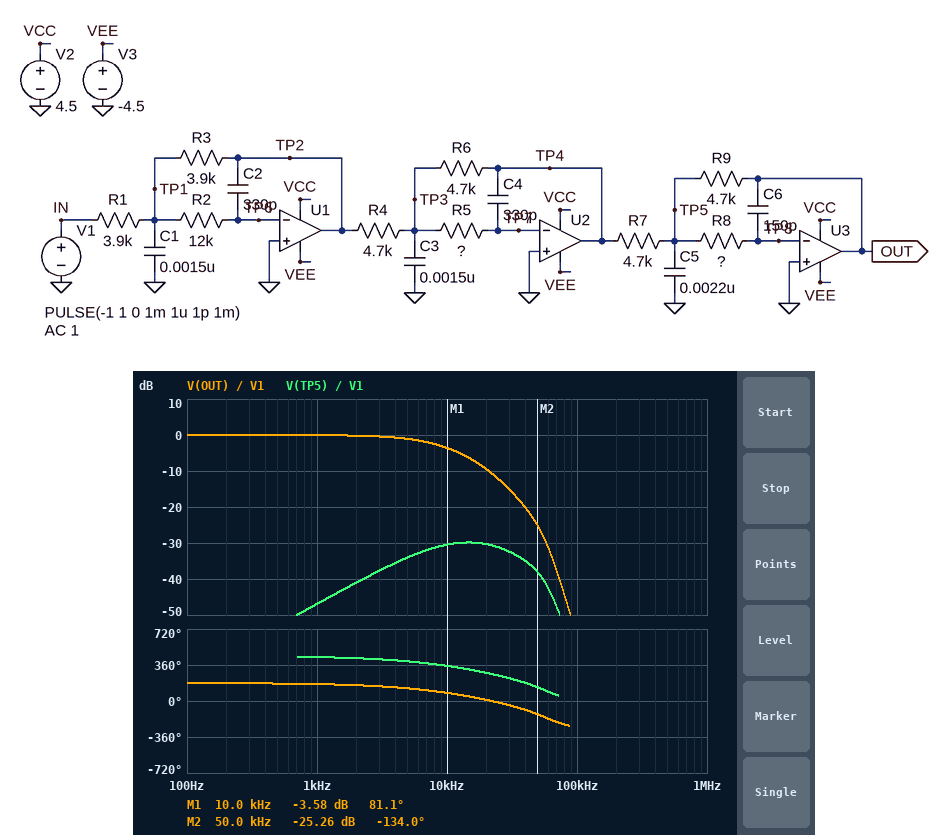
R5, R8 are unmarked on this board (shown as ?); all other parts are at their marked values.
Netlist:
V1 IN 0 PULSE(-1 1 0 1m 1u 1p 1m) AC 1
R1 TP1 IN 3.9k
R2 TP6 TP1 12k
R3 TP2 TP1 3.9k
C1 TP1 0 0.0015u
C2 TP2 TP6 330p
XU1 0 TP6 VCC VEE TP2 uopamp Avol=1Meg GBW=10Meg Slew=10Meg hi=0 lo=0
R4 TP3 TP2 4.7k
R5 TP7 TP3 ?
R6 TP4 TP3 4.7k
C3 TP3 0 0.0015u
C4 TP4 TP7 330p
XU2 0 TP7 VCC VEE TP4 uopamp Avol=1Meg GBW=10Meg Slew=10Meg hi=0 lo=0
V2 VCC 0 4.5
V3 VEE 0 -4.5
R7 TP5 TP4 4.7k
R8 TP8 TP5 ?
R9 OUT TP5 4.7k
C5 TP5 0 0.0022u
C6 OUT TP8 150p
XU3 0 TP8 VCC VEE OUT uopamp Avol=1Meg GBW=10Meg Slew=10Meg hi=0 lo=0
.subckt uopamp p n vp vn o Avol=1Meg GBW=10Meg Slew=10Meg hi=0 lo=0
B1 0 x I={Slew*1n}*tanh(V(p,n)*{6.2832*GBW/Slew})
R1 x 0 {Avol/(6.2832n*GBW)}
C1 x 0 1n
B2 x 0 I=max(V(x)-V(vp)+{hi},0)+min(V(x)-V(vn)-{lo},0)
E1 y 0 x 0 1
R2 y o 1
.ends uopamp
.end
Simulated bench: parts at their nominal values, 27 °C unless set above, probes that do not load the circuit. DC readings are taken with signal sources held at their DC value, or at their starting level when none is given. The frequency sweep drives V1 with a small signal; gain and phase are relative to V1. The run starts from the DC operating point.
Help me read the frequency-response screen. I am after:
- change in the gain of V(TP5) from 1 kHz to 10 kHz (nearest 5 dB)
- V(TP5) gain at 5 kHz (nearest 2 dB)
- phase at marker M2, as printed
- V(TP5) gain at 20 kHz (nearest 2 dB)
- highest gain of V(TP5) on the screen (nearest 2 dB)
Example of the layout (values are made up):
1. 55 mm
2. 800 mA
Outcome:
1. 15 dB
2. -34 dB
3. -134.0 deg
4. -30 dB
5. -30 dB
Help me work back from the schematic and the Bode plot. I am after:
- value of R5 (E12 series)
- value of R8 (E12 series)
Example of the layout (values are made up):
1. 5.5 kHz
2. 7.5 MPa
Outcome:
1. 27 kΩ
2. 4.7 kΩ
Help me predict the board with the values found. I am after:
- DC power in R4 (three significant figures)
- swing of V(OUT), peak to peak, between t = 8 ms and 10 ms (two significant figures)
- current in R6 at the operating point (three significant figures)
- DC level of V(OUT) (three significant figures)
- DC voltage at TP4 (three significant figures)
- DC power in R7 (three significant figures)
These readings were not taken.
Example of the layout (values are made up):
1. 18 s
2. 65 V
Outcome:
1. 213 µW
2. 1.8 V
3. 213 µA
4. 1.00 V
5. -1.00 V
6. 213 µW
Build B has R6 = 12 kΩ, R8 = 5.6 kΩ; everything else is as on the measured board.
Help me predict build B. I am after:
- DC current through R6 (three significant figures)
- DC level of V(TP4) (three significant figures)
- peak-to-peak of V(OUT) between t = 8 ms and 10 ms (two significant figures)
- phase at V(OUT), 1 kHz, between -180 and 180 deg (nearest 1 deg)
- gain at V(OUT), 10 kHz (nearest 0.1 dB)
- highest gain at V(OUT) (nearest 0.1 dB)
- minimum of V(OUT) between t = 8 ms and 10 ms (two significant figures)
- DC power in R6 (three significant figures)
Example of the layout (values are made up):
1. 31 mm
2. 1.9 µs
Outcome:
1. 213 µA
2. -2.55 V
3. 4.3 V
4. 163 deg
5. 0.6 dB
6. 8.1 dB
7. -2.3 V
8. 543 µW
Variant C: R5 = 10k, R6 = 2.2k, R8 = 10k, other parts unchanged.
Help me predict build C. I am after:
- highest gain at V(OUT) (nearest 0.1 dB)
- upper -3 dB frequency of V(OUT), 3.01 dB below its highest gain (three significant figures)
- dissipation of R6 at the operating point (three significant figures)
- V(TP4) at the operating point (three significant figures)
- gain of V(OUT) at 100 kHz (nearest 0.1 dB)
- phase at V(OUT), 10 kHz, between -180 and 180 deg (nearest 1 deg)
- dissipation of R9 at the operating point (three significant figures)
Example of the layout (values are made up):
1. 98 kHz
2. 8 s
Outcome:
1. -6.6 dB
2. 24.0 kHz
3. 99.6 µW
4. -468 mV
5. -55.4 dB
6. 113 deg
7. 46.6 µW
